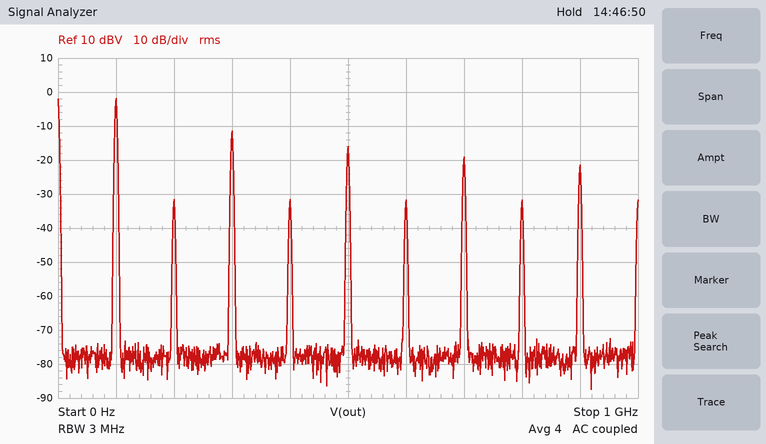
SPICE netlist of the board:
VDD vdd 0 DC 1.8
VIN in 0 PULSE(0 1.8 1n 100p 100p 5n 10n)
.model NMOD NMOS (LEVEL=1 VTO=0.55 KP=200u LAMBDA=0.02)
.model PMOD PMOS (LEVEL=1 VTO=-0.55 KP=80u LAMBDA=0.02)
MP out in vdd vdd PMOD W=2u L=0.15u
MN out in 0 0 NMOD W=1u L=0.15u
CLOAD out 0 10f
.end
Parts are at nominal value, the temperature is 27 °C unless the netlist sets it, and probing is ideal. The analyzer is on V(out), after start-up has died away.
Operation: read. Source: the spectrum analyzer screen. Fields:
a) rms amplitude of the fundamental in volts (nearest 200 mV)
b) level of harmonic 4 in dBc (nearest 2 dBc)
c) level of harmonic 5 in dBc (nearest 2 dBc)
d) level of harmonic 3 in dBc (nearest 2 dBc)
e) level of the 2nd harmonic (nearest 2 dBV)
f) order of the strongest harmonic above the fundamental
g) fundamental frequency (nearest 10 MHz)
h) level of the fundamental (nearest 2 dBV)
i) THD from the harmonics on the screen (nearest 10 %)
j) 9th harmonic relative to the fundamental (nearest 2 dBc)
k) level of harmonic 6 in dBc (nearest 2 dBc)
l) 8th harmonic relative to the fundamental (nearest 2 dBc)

800 mV
-30 dBc
-14 dBc
-10 dBc
-32 dBV
3
100 MHz
-2 dBV
40 %
-20 dBc
-30 dBc
-30 dBc
